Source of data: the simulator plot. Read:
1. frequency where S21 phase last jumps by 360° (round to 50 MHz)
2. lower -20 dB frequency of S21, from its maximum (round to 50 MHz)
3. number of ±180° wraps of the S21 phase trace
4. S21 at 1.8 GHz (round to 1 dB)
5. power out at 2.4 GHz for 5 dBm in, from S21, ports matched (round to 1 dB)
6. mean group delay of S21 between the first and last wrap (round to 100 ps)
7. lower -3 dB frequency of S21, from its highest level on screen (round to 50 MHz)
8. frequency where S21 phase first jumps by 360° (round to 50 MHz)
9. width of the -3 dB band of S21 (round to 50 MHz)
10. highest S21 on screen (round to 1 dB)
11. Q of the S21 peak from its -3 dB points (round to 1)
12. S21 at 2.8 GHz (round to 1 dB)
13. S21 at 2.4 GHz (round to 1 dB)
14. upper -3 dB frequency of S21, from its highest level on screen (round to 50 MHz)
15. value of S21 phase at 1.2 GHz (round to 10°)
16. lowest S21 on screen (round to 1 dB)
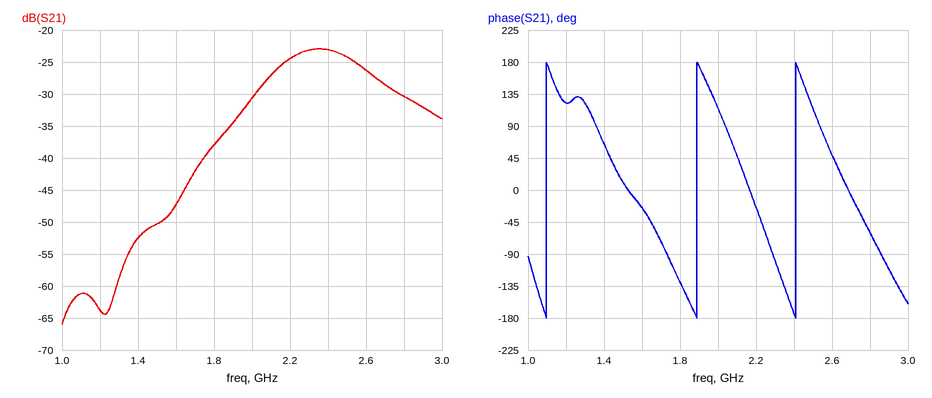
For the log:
2.40 GHz
1.70 GHz
3
-38 dB
-18 dBm
1.5 ns
2.15 GHz
1.10 GHz
450 MHz
-23 dB
5
-30 dB
-23 dB
2.60 GHz
120°
-66 dB
